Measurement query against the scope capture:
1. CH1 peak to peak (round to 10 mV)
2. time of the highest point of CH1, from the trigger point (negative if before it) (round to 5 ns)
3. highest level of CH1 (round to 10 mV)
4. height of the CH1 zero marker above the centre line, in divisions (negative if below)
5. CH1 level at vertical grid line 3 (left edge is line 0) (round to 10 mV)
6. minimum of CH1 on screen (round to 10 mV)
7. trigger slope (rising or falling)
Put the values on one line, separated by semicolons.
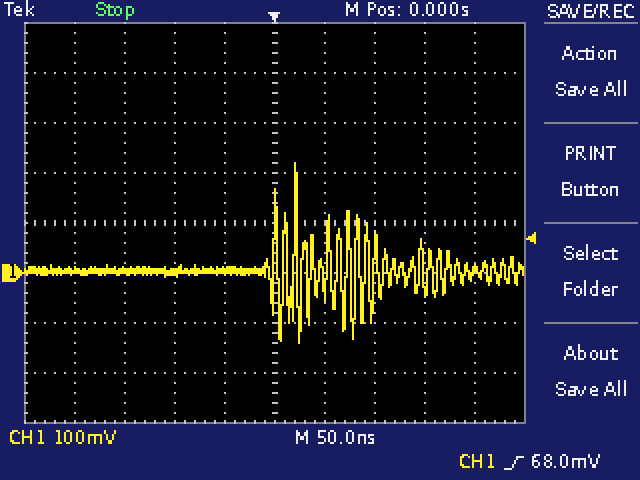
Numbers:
360 mV; +20 ns; 220 mV; -1.0 div; 0 mV; -140 mV; rising
